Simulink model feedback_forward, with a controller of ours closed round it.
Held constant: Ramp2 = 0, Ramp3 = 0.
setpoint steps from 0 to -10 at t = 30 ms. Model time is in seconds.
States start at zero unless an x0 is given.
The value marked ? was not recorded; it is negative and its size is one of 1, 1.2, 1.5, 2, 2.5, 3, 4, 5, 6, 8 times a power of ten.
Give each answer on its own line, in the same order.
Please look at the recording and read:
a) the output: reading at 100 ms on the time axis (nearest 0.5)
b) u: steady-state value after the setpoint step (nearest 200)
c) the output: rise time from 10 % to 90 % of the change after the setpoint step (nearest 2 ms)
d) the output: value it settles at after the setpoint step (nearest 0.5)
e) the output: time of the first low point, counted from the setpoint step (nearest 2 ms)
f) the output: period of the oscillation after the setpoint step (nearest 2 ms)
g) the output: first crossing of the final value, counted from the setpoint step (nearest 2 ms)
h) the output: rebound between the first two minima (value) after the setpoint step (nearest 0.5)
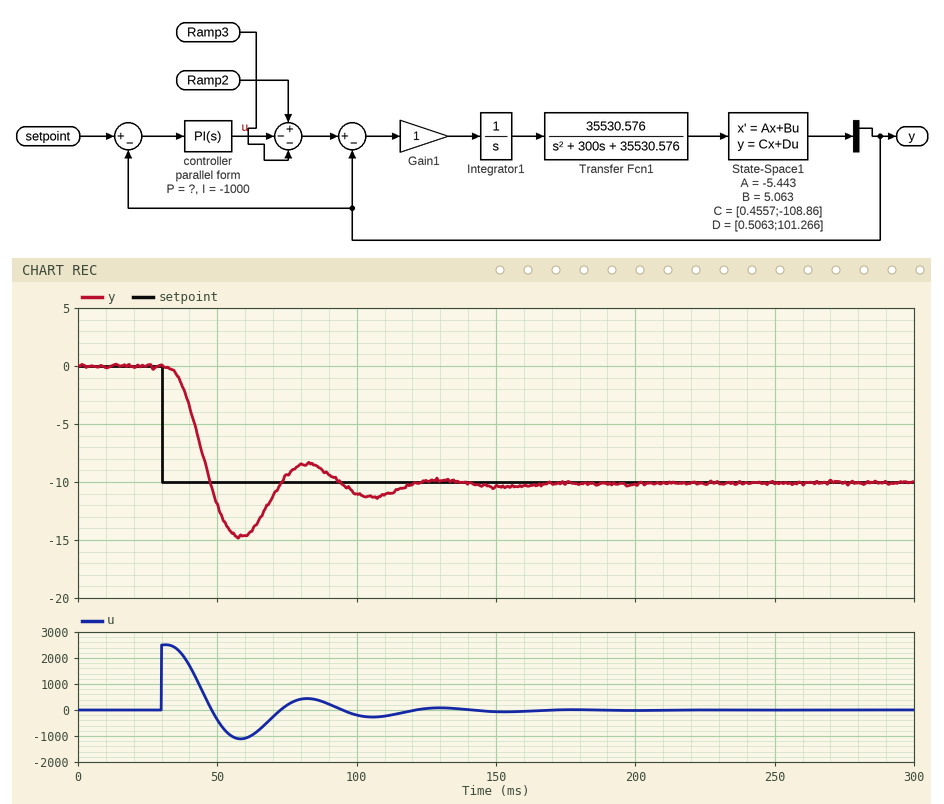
-11.0
0
10 ms
-10.0
28 ms
48 ms
18 ms
-8.5
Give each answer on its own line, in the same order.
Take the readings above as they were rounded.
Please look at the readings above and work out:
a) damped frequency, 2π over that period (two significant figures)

0.13 rad/ms
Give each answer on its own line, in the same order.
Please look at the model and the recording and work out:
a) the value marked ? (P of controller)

-250
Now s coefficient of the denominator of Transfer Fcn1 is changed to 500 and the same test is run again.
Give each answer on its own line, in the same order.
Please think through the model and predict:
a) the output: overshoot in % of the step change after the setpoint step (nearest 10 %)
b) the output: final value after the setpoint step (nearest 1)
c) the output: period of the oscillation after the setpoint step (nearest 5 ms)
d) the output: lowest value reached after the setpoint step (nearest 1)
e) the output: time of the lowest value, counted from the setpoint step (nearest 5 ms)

50 %
-10
65 ms
-15
35 ms
